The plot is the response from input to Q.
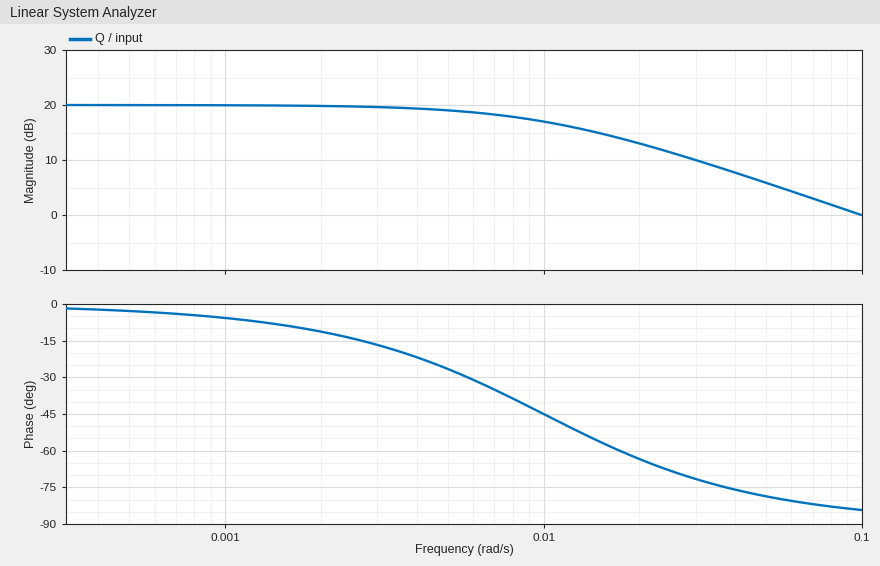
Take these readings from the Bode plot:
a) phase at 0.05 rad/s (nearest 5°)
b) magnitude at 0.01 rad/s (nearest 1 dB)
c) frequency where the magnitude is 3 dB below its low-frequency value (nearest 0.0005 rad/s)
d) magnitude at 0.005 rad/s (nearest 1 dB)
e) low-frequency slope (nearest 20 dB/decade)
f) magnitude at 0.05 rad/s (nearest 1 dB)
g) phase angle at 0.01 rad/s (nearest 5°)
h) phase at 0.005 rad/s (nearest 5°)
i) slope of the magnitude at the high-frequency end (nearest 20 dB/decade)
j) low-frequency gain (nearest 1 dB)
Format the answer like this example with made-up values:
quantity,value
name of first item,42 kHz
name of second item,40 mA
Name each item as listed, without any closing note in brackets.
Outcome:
quantity,value
phase at 0.05 rad/s,-80°
magnitude at 0.01 rad/s,17 dB
frequency where the magnitude is 3 dB below its low-frequency value,0.0100 rad/s
magnitude at 0.005 rad/s,19 dB
low-frequency slope,0 dB/decade
magnitude at 0.05 rad/s,6 dB
phase angle at 0.01 rad/s,-45°
phase at 0.005 rad/s,-25°
slope of the magnitude at the high-frequency end,-20 dB/decade
low-frequency gain,20 dB
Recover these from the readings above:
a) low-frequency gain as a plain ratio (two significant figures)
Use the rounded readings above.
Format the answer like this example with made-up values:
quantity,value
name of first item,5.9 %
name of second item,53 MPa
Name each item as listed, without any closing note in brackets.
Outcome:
quantity,value
low-frequency gain as a plain ratio,10
